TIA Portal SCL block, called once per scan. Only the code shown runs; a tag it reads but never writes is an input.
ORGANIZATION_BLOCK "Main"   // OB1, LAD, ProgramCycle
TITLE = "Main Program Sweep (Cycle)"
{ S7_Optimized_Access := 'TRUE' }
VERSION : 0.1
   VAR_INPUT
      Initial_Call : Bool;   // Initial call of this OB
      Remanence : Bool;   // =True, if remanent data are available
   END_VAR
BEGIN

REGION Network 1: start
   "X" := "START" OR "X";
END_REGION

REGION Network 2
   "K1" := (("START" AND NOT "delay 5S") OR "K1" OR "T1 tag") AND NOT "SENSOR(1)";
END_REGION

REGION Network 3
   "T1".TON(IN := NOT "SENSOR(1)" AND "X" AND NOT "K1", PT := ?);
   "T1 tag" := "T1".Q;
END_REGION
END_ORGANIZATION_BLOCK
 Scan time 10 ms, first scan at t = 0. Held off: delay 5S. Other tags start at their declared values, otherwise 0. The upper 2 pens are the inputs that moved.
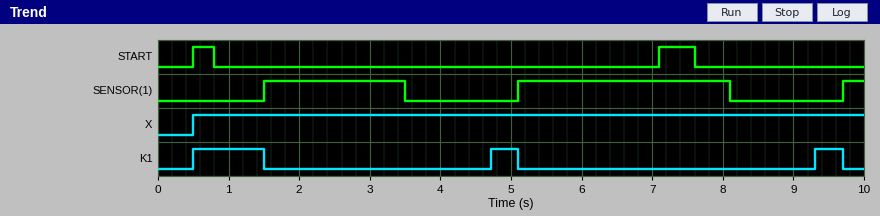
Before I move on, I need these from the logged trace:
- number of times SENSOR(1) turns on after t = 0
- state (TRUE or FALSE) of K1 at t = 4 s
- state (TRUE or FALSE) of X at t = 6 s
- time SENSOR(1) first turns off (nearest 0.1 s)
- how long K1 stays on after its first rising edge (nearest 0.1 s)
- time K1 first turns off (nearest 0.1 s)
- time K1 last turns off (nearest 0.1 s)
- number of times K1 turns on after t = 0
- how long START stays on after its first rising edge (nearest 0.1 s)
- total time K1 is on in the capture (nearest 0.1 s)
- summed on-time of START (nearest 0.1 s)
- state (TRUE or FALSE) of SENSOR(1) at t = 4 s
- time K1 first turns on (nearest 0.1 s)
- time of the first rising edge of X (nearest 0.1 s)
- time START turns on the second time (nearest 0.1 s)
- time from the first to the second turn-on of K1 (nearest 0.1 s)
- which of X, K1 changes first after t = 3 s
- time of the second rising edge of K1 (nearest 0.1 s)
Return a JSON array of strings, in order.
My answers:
["3", "FALSE", "TRUE", "3.5 s", "1.0 s", "1.5 s", "9.7 s", "3", "0.3 s", "1.8 s", "0.8 s", "FALSE", "0.5 s", "0.5 s", "7.1 s", "4.2 s", "K1", "4.7 s"]
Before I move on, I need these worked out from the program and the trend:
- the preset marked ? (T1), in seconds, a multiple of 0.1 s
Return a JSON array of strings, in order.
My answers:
["1.2 s"]
